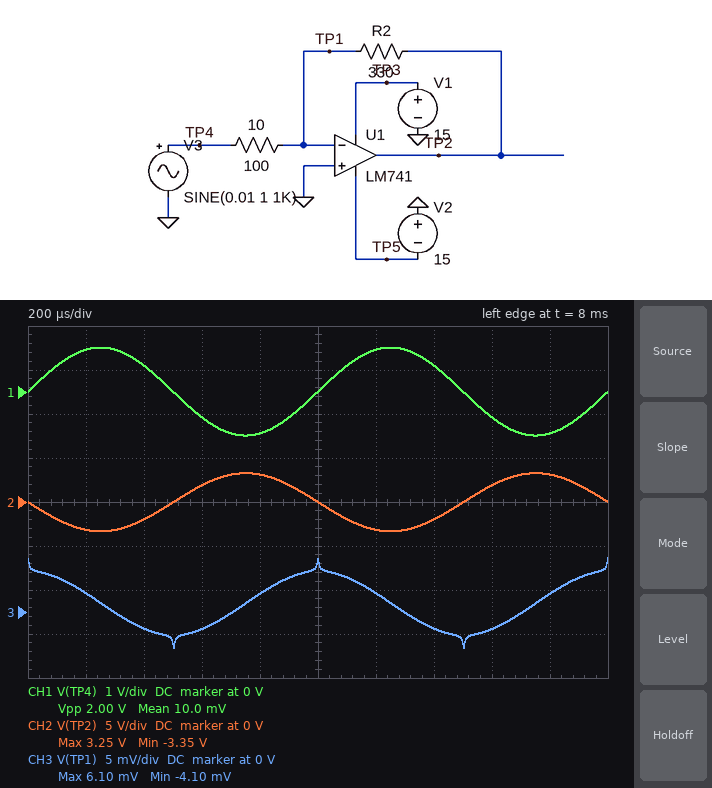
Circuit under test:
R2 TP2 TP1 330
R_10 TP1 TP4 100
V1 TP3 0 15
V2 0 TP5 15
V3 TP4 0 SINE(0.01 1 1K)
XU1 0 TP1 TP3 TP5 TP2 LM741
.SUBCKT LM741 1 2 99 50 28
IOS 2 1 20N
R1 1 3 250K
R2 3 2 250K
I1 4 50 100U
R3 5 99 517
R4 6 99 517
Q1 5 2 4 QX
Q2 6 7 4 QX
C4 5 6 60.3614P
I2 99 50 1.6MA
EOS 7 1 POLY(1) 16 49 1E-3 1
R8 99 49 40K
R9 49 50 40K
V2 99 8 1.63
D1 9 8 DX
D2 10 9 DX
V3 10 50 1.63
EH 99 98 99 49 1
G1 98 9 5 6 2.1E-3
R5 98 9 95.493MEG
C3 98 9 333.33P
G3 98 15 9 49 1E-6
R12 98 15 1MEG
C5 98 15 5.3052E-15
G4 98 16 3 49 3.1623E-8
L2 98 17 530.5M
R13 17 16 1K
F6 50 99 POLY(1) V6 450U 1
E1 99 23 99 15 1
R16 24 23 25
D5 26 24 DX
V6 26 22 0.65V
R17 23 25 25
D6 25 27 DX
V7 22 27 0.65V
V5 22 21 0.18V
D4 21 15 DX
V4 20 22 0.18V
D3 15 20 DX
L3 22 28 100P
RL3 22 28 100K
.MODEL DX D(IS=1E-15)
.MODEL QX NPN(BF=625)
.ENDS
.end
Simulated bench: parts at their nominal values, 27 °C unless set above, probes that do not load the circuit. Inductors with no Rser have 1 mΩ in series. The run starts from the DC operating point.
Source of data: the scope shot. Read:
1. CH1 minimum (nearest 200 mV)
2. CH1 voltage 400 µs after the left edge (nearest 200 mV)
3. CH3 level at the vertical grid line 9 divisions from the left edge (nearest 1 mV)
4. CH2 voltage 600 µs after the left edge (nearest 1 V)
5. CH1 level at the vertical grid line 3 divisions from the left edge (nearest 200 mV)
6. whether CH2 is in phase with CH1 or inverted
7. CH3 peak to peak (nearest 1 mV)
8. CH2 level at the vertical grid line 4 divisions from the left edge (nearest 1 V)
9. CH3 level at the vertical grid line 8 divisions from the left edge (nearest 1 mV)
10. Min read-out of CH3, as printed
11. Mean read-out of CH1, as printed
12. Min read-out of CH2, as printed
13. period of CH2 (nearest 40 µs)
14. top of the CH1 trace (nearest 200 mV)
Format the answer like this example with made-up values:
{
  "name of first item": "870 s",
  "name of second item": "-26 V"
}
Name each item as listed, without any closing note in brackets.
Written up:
{
  "CH1 minimum": "-1.0 V",
  "CH1 voltage 400 µs after the left edge": "600 mV",
  "CH3 level at the vertical grid line 9 divisions from the left edge": "2 mV",
  "CH2 voltage 600 µs after the left edge": "2 V",
  "CH1 level at the vertical grid line 3 divisions from the left edge": "-600 mV",
  "whether CH2 is in phase with CH1 or inverted": "inverted",
  "CH3 peak to peak": "10 mV",
  "CH2 level at the vertical grid line 4 divisions from the left edge": "3 V",
  "CH3 level at the vertical grid line 8 divisions from the left edge": "-2 mV",
  "Min read-out of CH3, as printed": "-4.10 mV",
  "Mean read-out of CH1, as printed": "10.0 mV",
  "Min read-out of CH2, as printed": "-3.35 V",
  "period of CH2": "1.00 ms",
  "top of the CH1 trace": "1.0 V"
}
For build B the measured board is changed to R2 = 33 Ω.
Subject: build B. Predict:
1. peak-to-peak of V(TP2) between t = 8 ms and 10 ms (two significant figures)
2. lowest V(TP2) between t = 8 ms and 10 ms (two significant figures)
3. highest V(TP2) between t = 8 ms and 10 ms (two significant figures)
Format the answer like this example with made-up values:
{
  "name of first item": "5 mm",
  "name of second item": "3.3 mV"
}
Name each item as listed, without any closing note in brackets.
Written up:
{
  "peak-to-peak of V(TP2) between t = 8 ms and 10 ms": "660 mV",
  "lowest V(TP2) between t = 8 ms and 10 ms": "-330 mV",
  "highest V(TP2) between t = 8 ms and 10 ms": "330 mV"
}
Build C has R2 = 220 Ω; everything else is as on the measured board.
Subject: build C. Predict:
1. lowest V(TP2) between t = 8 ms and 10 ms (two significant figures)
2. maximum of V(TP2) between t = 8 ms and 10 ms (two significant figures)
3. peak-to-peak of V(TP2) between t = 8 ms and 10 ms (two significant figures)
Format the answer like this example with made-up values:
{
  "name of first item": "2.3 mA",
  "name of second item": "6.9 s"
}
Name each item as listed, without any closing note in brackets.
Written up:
{
  "lowest V(TP2) between t = 8 ms and 10 ms": "-2.2 V",
  "maximum of V(TP2) between t = 8 ms and 10 ms": "2.2 V",
  "peak-to-peak of V(TP2) between t = 8 ms and 10 ms": "4.4 V"
}
